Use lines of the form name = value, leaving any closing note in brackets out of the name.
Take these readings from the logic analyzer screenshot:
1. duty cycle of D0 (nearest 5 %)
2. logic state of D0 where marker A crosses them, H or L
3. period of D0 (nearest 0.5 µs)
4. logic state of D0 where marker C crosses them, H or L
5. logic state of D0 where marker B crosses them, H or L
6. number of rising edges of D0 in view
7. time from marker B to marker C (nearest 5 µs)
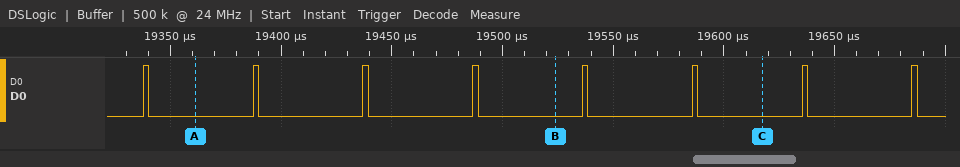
duty cycle of D0 = 5 %
logic state of D0 where marker A crosses them, H or L = D0=L
period of D0 = 49.5 µs
logic state of D0 where marker C crosses them, H or L = D0=L
logic state of D0 where marker B crosses them, H or L = D0=L
number of rising edges of D0 in view = 8
time from marker B to marker C = 95 µs
